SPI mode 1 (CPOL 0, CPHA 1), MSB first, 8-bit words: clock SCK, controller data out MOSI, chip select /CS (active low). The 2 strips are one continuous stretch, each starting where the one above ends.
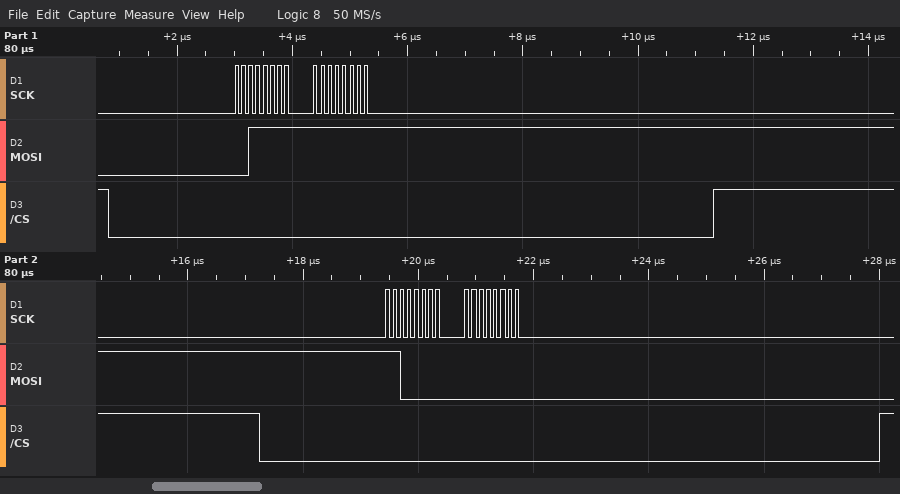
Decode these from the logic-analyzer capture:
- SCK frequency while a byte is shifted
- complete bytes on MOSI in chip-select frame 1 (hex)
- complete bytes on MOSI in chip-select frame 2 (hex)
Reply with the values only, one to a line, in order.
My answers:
8 MHz
0x3F 0xFF
0xC0 0x00
